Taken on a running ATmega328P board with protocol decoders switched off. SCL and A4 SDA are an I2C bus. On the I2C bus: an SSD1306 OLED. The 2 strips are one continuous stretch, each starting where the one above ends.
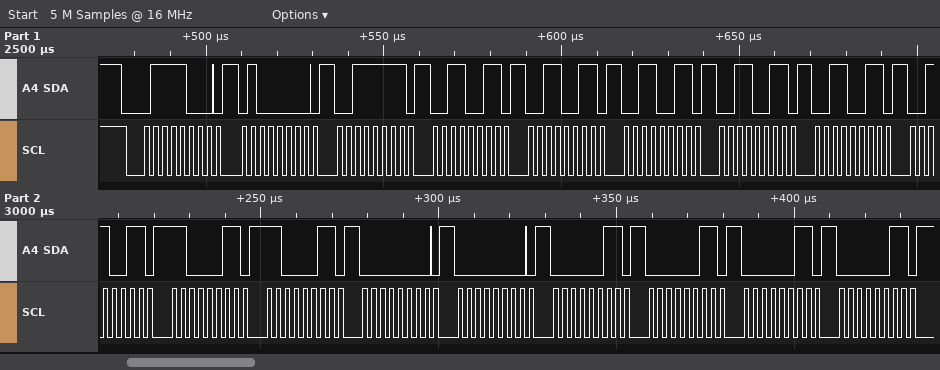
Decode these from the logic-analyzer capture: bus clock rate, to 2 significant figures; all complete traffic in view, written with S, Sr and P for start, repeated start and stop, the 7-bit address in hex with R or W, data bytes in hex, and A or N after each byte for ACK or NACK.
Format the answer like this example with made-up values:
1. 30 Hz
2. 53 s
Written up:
1. 400 kHz
2. S 3CW A 40 A 3F A 33 A 33 A 33 A 33 A 33 A 33 A C3 A C3 A 00 A 00 A 03 A 03 A 03 A 03 A
